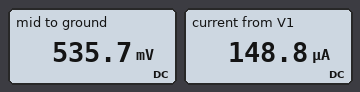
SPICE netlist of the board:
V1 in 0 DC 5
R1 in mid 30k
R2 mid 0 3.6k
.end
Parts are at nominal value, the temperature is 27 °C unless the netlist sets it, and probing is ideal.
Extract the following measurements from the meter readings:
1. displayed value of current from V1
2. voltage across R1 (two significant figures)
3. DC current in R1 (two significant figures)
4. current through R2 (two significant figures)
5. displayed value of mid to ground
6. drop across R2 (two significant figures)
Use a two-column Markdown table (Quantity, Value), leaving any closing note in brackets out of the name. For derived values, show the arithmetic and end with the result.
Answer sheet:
| Quantity | Value |
|---|---|
| displayed value of current from V1 | 148.8 µA |
| voltage across R1 | 5 V - 535.7 mV = 4.5 V |
| DC current in R1 | (5 V - 535.7 mV) / 30 kΩ = 150 µA |
| current through R2 | (535.7 mV) / 3.6 kΩ = 150 µA |
| displayed value of mid to ground | 535.7 mV |
| drop across R2 | 535.7 mV = 540 mV |
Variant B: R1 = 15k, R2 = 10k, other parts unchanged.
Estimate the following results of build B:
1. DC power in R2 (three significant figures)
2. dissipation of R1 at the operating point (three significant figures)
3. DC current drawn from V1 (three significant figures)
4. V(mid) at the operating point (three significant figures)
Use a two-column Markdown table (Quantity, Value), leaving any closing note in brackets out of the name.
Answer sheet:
| Quantity | Value |
|---|---|
| DC power in R2 | 400 µW |
| dissipation of R1 at the operating point | 600 µW |
| DC current drawn from V1 | 200 µA |
| V(mid) at the operating point | 2.00 V |
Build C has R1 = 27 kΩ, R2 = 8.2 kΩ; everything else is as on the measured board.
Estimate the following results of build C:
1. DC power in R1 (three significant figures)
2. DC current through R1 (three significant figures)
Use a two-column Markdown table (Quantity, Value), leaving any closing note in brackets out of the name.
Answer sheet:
| Quantity | Value |
|---|---|
| DC power in R1 | 545 µW |
| DC current through R1 | 142 µA |
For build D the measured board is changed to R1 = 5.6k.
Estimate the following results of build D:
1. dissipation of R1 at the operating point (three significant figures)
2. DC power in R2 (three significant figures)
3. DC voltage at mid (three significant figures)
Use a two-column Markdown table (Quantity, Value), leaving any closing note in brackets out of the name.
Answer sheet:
| Quantity | Value |
|---|---|
| dissipation of R1 at the operating point | 1.65 mW |
| DC power in R2 | 1.06 mW |
| DC voltage at mid | 1.96 V |
